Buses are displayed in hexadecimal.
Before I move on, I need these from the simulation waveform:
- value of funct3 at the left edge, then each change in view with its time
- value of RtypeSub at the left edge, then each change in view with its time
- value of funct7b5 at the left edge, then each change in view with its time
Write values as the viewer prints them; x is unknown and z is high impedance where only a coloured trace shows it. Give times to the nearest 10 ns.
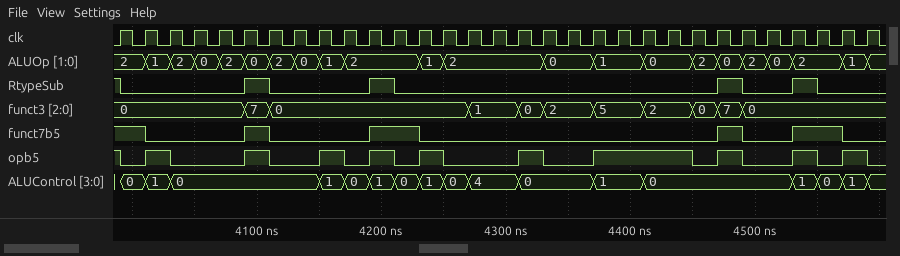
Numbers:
0, 7 at 4090 ns, 0 at 4110 ns, 1 at 4270 ns, 0 at 4310 ns, 2 at 4330 ns, 5 at 4370 ns, 2 at 4410 ns, 0 at 4450 ns, 7 at 4470 ns, 0 at 4490 ns
1, 0 at 3990 ns, 1 at 4090 ns, 0 at 4110 ns, 1 at 4190 ns, 0 at 4210 ns, 1 at 4470 ns, 0 at 4490 ns, 1 at 4530 ns, 0 at 4550 ns
1, 0 at 4010 ns, 1 at 4090 ns, 0 at 4110 ns, 1 at 4190 ns, 0 at 4230 ns, 1 at 4470 ns, 0 at 4490 ns, 1 at 4530 ns, 0 at 4570 ns
